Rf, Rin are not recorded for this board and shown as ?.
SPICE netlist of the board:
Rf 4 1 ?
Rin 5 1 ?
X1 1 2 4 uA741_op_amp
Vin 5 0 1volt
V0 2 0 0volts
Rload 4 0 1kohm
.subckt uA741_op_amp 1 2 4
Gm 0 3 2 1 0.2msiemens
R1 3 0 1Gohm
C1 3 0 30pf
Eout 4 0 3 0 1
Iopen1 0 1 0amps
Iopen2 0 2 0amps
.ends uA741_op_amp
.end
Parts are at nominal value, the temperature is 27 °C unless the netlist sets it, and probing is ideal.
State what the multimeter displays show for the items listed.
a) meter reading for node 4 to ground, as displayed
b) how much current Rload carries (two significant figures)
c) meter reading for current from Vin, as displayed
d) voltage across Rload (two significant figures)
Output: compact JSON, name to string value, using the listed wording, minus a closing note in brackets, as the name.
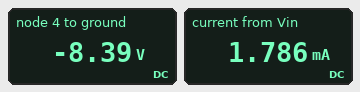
{"meter reading for node 4 to ground, as displayed": "-8.39 V", "how much current Rload carries": "8.4 mA", "meter reading for current from Vin, as displayed": "1.786 mA", "voltage across Rload": "8.4 V"}
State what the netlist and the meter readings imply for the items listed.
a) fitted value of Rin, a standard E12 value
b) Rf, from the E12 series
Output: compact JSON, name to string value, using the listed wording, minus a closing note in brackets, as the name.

{"fitted value of Rin, a standard E12 value": "560 Ω", "Rf, from the E12 series": "4.7 kΩ"}
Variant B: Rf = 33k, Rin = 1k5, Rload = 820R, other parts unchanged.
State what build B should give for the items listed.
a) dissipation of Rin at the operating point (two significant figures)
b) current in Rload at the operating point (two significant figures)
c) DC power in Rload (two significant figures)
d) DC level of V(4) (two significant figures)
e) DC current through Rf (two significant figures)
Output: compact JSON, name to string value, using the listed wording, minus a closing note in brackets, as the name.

{"dissipation of Rin at the operating point": "670 µW", "current in Rload at the operating point": "27 mA", "DC power in Rload": "590 mW", "DC level of V(4)": "-22 V", "DC current through Rf": "670 µA"}
